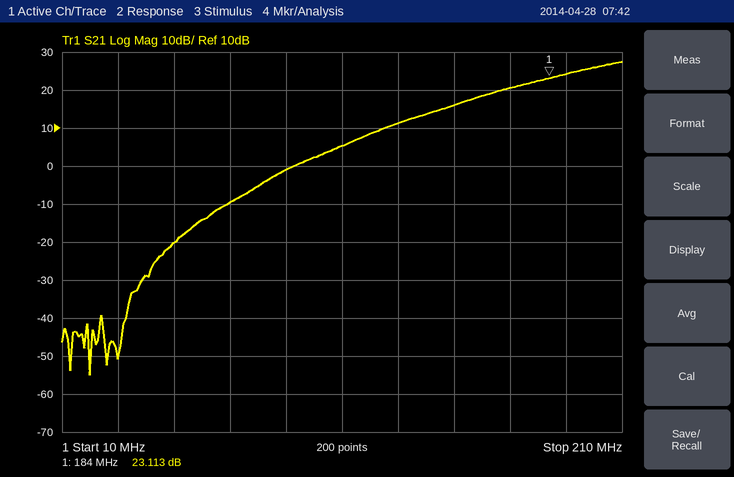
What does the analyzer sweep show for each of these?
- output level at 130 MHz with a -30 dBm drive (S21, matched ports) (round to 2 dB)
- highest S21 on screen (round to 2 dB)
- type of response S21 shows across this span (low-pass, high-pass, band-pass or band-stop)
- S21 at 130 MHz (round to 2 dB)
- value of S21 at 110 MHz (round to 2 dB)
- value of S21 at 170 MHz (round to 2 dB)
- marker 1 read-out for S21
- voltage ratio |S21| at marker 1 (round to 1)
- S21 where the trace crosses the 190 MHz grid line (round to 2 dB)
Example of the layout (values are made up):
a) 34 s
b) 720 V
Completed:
a) -18 dBm
b) 28 dB
c) high-pass
d) 12 dB
e) 6 dB
f) 20 dB
g) 23.113 dB
h) 14
i) 24 dB
